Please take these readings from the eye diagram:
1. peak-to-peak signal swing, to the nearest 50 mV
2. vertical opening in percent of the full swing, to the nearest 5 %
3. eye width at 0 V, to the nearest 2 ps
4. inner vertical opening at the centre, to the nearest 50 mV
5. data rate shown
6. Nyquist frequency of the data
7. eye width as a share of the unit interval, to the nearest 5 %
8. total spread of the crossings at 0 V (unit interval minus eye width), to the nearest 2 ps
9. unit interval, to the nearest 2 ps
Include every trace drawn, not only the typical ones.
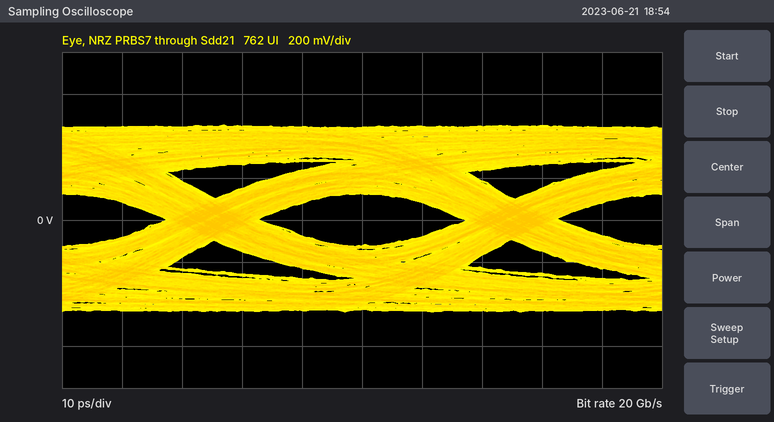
900 mV
30 %
34 ps
250 mV
20 Gb/s
10 GHz
70 %
16 ps
50 ps
